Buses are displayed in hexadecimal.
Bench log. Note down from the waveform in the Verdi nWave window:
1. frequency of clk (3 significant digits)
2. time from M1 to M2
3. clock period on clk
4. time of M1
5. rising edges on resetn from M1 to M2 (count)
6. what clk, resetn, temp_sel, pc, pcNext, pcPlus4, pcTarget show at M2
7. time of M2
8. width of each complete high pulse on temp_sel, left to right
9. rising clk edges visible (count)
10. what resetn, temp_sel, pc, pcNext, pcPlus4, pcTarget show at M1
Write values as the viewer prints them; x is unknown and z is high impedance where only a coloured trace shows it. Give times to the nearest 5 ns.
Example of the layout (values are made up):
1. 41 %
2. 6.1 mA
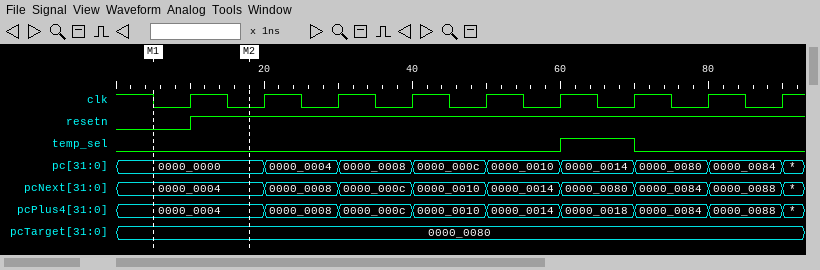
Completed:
1. 100 MHz
2. 15 ns
3. 10 ns
4. 5 ns
5. 1
6. clk=0, resetn=1, temp_sel=0, pc=0000_0000, pcNext=0000_0004, pcPlus4=0000_0004, pcTarget=0000_0080
7. 20 ns
8. 10 ns
9. 9
10. resetn=0, temp_sel=0, pc=0000_0000, pcNext=0000_0004, pcPlus4=0000_0004, pcTarget=0000_0080
